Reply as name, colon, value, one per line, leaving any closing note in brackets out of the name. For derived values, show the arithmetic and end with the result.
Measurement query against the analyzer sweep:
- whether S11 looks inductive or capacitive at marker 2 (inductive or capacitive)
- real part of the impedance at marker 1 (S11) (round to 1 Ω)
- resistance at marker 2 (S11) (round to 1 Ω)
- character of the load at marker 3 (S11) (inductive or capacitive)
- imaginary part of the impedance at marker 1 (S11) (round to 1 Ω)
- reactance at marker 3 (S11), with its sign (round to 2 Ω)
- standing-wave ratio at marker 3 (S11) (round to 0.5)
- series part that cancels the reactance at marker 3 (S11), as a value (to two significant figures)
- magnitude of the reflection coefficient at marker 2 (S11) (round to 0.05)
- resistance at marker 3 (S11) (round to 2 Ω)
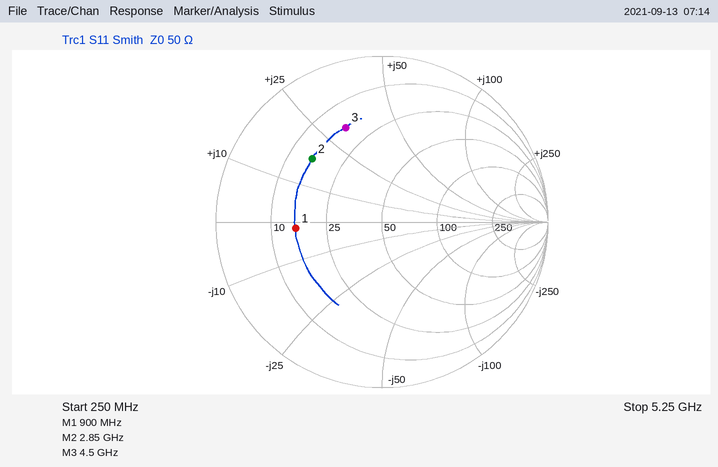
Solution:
whether S11 looks inductive or capacitive at marker 2: inductive
real part of the impedance at marker 1 (S11): 16 Ω
resistance at marker 2 (S11): 16 Ω
character of the load at marker 3 (S11): inductive
imaginary part of the impedance at marker 1 (S11): -2 Ω
reactance at marker 3 (S11), with its sign: +32 Ω
standing-wave ratio at marker 3 (S11): 4.0
series part that cancels the reactance at marker 3 (S11), as a value: C = 1/(2π × 4.5 GHz × 32 Ω) ≈ 1.1 pF
magnitude of the reflection coefficient at marker 2 (S11): 0.55
resistance at marker 3 (S11): 18 Ω
